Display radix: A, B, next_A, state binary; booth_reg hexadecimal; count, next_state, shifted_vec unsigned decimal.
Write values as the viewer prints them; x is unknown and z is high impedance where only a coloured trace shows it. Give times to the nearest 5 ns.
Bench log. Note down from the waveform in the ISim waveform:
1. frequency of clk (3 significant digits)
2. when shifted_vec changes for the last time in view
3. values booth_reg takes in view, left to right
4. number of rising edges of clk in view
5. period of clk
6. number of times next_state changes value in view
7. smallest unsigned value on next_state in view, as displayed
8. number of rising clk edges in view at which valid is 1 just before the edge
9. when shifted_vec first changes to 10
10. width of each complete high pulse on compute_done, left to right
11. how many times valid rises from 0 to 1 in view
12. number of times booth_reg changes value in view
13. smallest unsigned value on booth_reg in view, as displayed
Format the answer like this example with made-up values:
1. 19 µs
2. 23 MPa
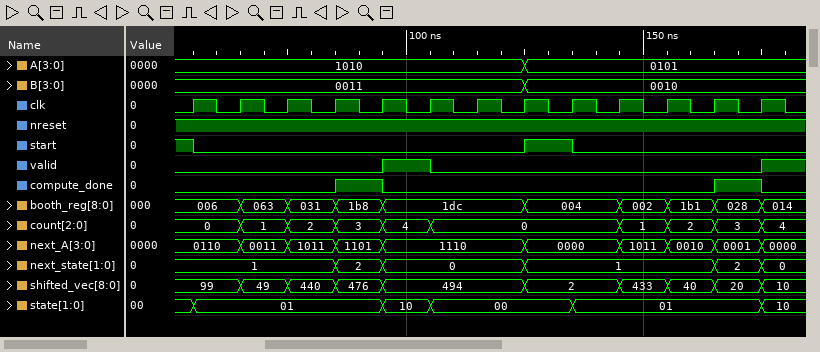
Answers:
1. 100 MHz
2. 175 ns
3. 006, 063, 031, 1b8, 1dc, 004, 002, 1b1, 028, 014
4. 13
5. 10 ns
6. 5
7. 0
8. 1
9. 175 ns
10. 10 ns, 10 ns
11. 2
12. 9
13. 002
